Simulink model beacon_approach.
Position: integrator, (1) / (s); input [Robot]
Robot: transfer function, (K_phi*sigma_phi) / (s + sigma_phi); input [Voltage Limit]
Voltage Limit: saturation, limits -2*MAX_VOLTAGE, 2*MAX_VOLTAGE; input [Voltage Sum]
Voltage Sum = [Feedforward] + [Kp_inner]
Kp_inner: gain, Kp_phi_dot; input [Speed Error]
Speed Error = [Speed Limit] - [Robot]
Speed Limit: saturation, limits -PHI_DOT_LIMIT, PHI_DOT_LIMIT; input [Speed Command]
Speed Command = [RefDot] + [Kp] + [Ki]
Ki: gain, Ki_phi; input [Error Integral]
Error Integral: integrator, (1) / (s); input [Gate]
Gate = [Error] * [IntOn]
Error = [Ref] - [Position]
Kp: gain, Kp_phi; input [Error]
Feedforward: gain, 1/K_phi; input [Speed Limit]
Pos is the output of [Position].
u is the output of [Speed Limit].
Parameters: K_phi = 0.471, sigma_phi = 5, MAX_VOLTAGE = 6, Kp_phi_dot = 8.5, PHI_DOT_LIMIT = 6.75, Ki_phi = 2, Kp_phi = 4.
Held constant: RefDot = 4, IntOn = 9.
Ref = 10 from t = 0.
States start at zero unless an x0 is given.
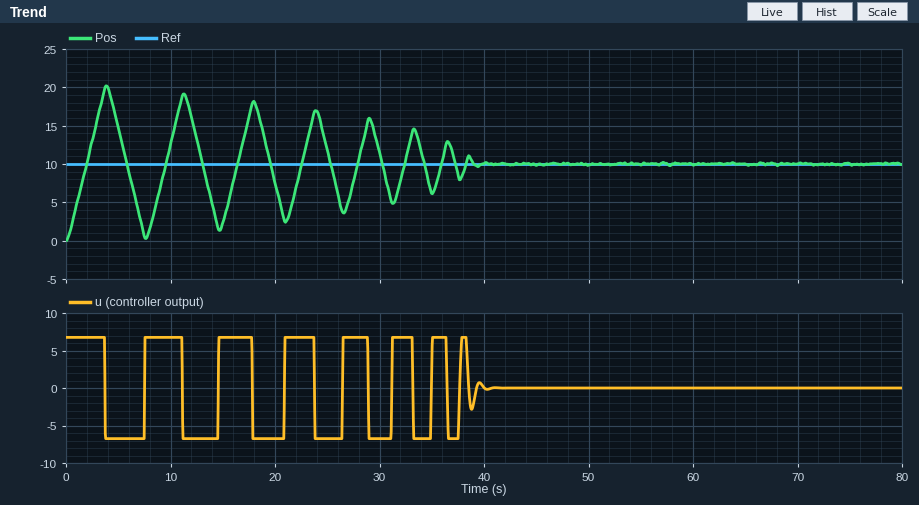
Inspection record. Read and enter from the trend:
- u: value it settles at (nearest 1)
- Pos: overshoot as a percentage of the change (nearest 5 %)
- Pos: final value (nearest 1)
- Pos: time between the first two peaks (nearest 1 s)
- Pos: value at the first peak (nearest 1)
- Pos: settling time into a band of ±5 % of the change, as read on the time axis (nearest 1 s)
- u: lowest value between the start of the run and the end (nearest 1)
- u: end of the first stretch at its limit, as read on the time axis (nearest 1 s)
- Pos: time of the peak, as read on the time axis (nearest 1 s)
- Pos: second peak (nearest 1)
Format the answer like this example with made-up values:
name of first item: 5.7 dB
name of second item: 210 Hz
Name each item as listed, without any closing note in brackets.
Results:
u: value it settles at: 0
Pos: overshoot as a percentage of the change: 100 %
Pos: final value: 10
Pos: time between the first two peaks: 7 s
Pos: value at the first peak: 20
Pos: settling time into a band of ±5 % of the change, as read on the time axis: 39 s
u: lowest value between the start of the run and the end: -7
u: end of the first stretch at its limit, as read on the time axis: 4 s
Pos: time of the peak, as read on the time axis: 4 s
Pos: second peak: 19
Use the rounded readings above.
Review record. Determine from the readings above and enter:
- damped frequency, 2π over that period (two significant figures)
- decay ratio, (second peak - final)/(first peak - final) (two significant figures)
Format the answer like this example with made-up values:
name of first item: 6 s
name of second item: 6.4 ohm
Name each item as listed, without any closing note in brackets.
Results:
damped frequency, 2π over that period: 0.90 rad/s
decay ratio, (second peak - final)/(first peak - final): 0.90
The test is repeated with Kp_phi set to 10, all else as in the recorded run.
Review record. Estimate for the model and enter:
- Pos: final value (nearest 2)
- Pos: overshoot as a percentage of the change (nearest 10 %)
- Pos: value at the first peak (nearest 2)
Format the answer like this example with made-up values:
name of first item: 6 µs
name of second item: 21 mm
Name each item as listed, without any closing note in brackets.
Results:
Pos: final value: 10
Pos: overshoot as a percentage of the change: 90 %
Pos: value at the first peak: 18
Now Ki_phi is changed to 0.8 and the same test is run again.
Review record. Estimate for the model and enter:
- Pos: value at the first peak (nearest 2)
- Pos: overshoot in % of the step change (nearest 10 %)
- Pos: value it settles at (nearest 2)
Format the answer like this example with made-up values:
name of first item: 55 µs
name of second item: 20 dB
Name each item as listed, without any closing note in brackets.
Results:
Pos: value at the first peak: 18
Pos: overshoot in % of the step change: 90 %
Pos: value it settles at: 10
